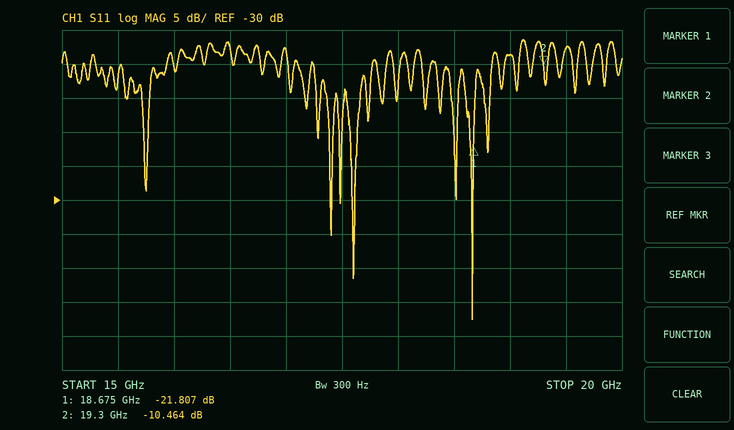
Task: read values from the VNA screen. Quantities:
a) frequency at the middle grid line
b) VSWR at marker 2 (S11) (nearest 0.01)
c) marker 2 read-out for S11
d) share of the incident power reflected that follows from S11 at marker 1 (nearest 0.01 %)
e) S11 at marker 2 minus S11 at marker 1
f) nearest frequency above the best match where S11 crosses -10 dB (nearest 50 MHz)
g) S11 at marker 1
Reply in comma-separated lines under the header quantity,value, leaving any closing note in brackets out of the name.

quantity,value
frequency at the middle grid line,17.5 GHz
VSWR at marker 2 (S11),1.86
marker 2 read-out for S11,-10.464 dB
share of the incident power reflected that follows from S11 at marker 1,0.66 %
S11 at marker 2 minus S11 at marker 1,11.343 dB
nearest frequency above the best match where S11 crosses -10 dB,18.85 GHz
S11 at marker 1,-21.807 dB
